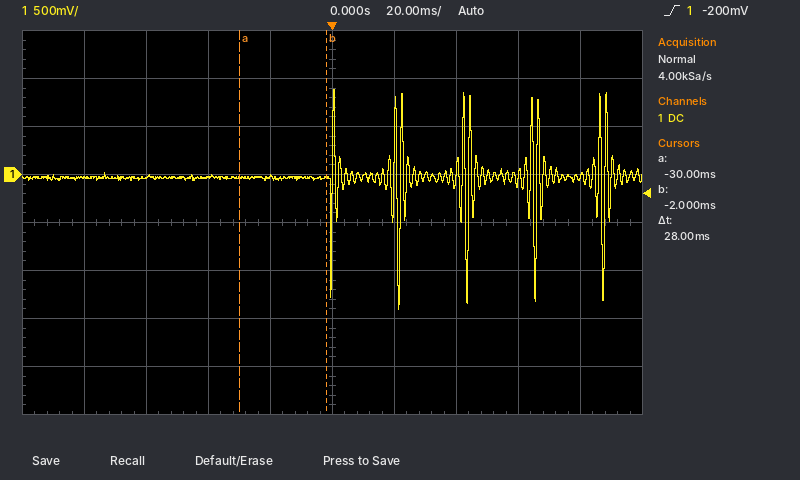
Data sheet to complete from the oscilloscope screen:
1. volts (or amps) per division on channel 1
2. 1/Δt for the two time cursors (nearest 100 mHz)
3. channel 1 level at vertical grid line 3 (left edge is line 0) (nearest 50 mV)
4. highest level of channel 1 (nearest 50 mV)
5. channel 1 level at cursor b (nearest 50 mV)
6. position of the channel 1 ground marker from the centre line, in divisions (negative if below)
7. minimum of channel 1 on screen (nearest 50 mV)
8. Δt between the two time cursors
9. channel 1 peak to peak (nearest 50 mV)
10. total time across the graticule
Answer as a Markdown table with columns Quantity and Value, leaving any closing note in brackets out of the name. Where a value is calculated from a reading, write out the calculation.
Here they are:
| Quantity | Value |
|---|---|
| volts (or amps) per division on channel 1 | 500 mV |
| 1/Δt for the two time cursors | 1 / 28 ms ≈ 35.7 Hz |
| channel 1 level at vertical grid line 3 (left edge is line 0) | -50 mV |
| highest level of channel 1 | 900 mV |
| channel 1 level at cursor b | -50 mV |
| position of the channel 1 ground marker from the centre line, in divisions | +1.0 div |
| minimum of channel 1 on screen | -1.40 V |
| Δt between the two time cursors | 28 ms |
| channel 1 peak to peak | 900 mV − (-1.40 V) = 2.30 V |
| total time across the graticule | 200 ms |
